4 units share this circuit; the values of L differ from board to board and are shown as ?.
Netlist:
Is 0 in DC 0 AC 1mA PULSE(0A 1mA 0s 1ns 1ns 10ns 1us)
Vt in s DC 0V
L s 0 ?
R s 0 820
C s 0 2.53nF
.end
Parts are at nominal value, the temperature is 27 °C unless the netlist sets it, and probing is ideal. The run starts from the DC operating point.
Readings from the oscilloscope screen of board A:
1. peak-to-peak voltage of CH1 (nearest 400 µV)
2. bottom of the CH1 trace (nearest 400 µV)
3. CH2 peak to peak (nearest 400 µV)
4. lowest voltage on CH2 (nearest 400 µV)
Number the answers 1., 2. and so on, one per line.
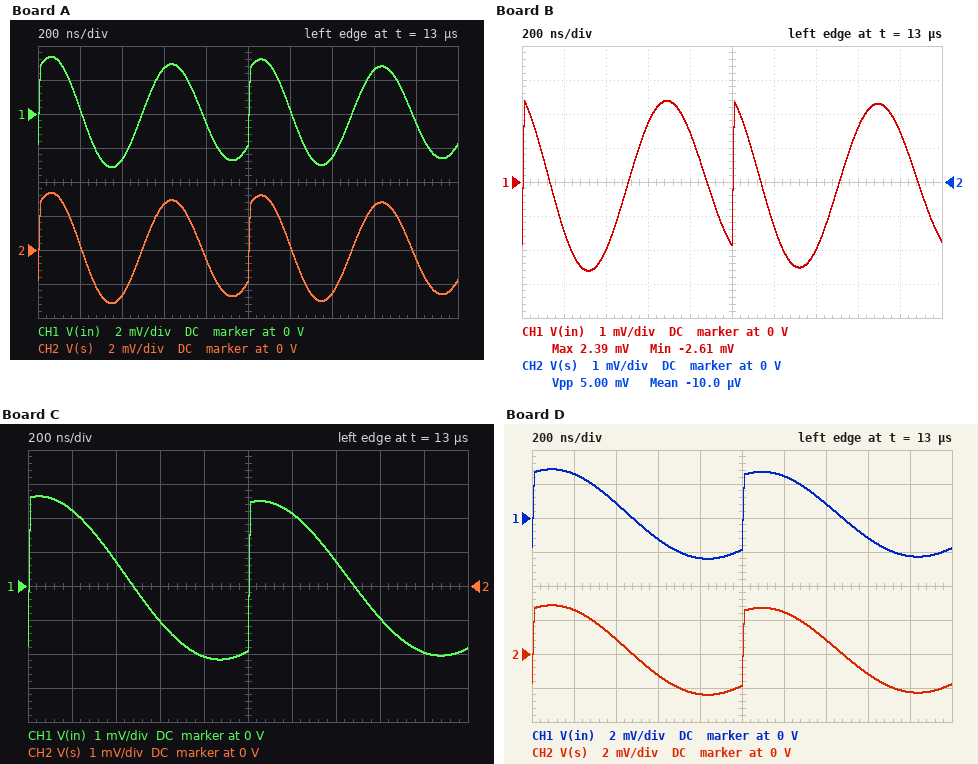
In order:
1. 6.4 mV
2. -3.2 mV
3. 6.4 mV
4. -3.2 mV
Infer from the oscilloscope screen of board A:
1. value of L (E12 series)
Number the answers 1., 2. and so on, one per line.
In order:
1. 3.3 µH
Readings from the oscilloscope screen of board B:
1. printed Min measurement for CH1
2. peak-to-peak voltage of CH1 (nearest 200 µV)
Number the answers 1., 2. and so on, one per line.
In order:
1. -2.61 mV
2. 5.0 mV
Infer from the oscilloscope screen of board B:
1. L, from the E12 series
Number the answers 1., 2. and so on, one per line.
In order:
1. 5.6 µH
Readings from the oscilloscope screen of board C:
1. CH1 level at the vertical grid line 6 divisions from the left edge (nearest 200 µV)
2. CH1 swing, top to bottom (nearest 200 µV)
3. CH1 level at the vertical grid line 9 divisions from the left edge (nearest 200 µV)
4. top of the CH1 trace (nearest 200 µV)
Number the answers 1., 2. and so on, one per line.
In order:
1. 2.2 mV
2. 4.8 mV
3. -2.0 mV
4. 2.6 mV
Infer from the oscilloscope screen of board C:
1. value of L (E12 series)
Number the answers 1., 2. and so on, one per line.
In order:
1. 27 µH
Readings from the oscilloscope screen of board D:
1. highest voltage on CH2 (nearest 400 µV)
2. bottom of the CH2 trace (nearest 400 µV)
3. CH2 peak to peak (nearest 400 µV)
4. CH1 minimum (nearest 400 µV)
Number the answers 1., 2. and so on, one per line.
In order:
1. 2.8 mV
2. -2.4 mV
3. 5.2 mV
4. -2.4 mV
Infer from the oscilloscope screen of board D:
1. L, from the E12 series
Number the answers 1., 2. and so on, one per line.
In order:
1. 22 µH
